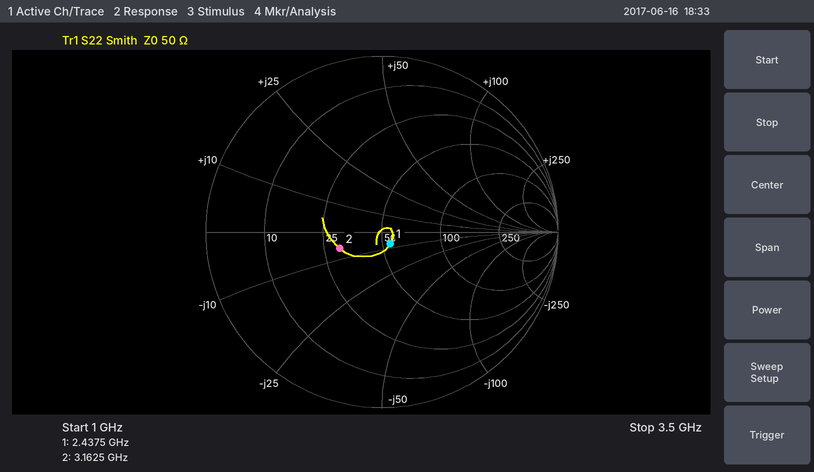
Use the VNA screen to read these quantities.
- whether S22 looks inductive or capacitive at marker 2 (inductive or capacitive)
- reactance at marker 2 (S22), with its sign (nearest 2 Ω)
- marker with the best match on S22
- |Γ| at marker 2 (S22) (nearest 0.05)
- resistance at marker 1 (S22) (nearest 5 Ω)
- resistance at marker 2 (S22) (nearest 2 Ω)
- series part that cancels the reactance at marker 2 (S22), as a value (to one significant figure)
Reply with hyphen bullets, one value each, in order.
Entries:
- capacitive
- -6 Ω
- marker 1
- 0.25
- 55 Ω
- 30 Ω
- 300 pH
